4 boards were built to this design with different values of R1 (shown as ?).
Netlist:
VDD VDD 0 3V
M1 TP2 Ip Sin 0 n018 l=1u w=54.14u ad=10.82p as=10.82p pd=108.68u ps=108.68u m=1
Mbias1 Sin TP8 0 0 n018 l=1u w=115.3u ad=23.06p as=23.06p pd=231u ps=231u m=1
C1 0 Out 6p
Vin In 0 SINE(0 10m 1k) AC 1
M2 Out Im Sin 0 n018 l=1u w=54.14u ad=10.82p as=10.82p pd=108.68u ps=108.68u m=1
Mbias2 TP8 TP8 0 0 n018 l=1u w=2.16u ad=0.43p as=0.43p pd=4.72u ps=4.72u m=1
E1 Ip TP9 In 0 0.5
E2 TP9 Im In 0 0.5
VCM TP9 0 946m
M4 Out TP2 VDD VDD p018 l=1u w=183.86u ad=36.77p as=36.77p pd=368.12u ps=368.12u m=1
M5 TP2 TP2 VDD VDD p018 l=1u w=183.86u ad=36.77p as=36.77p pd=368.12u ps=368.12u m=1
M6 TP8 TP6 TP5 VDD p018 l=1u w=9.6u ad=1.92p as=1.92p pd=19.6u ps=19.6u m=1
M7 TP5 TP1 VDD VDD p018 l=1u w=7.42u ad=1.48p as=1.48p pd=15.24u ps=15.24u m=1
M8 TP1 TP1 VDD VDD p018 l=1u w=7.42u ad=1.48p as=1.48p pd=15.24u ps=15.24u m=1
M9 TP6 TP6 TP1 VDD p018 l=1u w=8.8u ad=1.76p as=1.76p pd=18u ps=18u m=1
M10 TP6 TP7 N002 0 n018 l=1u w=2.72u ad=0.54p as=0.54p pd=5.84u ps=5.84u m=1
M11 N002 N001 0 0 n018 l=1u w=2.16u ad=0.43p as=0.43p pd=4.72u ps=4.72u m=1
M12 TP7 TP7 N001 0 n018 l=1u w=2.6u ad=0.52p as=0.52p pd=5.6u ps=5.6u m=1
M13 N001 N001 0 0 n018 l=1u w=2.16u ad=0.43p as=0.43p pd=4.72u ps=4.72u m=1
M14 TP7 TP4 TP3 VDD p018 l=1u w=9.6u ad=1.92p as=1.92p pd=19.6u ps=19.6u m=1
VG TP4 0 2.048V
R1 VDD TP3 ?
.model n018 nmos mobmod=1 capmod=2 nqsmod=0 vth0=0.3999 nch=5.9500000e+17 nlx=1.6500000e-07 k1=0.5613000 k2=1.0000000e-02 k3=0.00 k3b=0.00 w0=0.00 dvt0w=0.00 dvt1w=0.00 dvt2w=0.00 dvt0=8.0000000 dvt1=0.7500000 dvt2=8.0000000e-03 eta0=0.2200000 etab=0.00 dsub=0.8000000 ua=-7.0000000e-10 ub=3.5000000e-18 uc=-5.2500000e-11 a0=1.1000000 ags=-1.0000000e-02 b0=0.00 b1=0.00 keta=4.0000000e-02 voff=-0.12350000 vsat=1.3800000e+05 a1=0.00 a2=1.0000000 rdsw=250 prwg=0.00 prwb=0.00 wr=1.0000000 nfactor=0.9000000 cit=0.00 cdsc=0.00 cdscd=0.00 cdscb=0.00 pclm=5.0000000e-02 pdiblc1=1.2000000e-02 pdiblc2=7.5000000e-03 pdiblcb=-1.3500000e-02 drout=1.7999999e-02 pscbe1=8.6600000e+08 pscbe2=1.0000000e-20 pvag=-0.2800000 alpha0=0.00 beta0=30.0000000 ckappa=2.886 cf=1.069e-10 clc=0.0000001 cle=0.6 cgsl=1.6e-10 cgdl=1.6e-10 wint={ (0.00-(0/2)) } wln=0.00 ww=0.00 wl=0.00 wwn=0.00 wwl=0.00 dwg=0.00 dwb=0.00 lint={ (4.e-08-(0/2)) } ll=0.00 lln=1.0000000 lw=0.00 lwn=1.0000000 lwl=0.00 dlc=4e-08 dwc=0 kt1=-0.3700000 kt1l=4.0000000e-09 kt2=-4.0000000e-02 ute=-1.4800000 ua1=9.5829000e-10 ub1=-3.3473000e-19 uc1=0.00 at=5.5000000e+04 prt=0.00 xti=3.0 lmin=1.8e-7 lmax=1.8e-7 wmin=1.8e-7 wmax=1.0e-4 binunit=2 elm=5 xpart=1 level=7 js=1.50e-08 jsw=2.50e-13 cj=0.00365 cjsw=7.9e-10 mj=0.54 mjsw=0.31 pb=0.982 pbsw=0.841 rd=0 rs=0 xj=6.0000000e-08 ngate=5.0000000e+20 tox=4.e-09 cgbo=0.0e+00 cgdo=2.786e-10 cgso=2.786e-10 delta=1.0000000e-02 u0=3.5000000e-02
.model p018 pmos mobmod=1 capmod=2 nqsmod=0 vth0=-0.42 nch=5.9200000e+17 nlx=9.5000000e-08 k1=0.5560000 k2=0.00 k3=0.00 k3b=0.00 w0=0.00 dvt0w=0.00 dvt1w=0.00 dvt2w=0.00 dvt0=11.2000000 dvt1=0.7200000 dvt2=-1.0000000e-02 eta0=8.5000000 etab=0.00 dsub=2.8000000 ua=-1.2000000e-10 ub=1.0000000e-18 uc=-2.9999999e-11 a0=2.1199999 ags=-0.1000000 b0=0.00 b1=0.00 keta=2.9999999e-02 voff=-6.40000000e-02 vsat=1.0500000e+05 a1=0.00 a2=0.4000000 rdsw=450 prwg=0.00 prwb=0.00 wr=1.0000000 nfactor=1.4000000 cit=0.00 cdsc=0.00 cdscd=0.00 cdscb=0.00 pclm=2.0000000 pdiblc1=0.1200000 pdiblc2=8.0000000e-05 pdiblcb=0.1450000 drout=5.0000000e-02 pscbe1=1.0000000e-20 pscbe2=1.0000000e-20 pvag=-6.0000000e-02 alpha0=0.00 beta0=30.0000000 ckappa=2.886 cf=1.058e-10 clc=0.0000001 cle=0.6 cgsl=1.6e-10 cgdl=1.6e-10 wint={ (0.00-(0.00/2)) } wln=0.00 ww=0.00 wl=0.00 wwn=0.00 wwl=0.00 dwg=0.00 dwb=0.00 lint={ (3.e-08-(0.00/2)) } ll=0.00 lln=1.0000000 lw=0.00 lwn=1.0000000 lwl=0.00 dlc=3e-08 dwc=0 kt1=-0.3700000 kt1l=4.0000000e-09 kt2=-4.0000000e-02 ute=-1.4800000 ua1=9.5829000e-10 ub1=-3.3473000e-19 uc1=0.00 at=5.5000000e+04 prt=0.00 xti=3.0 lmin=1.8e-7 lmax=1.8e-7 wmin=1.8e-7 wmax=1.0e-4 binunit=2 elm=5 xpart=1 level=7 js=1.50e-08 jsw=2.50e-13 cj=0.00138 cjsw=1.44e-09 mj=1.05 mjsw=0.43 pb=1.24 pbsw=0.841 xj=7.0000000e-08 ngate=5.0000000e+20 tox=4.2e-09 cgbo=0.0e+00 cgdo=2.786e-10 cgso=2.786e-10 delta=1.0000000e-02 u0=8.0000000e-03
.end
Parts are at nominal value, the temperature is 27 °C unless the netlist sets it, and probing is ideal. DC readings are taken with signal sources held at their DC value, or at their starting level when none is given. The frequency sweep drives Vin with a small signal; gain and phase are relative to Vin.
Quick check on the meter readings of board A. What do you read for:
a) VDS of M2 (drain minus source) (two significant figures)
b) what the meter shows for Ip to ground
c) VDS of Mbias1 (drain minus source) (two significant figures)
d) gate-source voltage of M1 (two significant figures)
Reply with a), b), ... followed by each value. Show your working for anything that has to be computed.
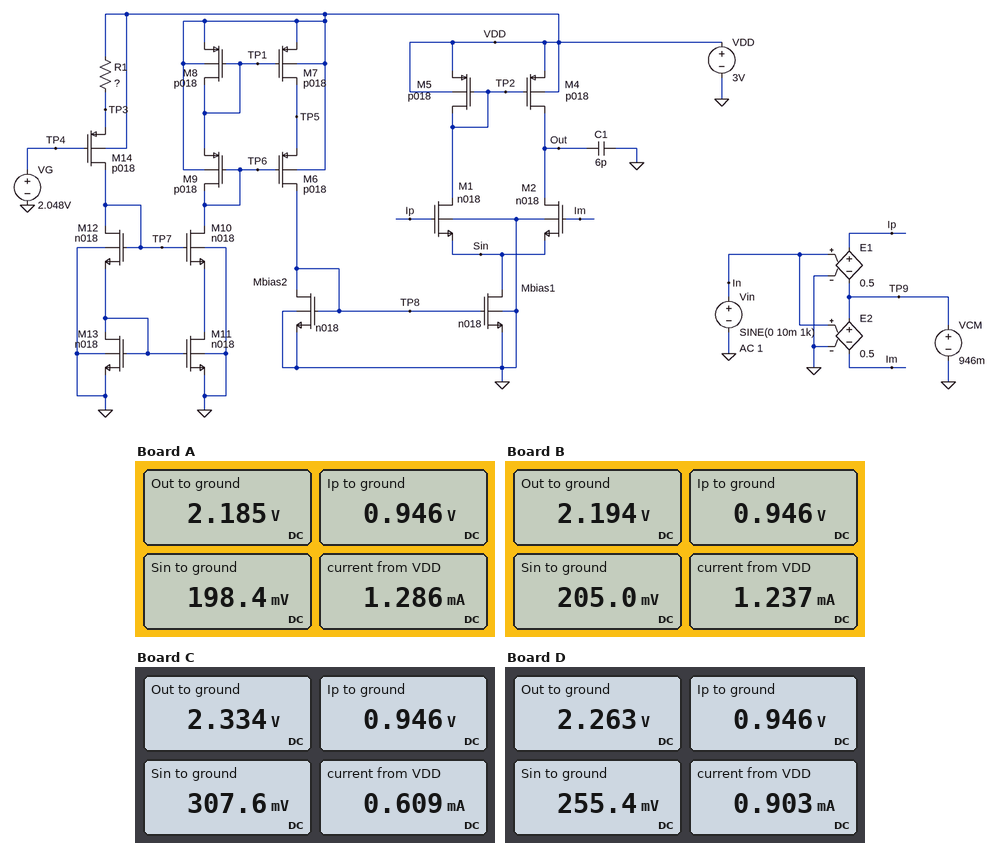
a) 2.185 V - 198.4 mV = 2.0 V
b) 0.946 V
c) 198.4 mV = 200 mV
d) 946 mV - 198.4 mV = 750 mV
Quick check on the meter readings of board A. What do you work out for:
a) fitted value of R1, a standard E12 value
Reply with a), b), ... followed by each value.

a) 6.8 kΩ
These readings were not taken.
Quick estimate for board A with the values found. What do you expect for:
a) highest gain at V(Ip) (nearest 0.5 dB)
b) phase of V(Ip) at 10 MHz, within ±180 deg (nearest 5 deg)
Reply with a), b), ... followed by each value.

a) -6.0 dB
b) 0 deg
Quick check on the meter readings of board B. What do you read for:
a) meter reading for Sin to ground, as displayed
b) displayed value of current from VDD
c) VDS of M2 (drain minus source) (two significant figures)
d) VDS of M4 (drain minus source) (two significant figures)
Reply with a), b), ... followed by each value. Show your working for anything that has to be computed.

a) 205.0 mV
b) 1.237 mA
c) 2.194 V - 205 mV = 2.0 V
d) 2.194 V - 3 V = -810 mV
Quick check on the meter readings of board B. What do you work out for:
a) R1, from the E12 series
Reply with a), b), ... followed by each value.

a) 8.2 kΩ
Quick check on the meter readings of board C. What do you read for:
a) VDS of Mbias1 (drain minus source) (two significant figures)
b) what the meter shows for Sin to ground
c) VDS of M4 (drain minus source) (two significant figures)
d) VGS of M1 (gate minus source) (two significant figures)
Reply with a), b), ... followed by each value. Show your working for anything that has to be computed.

a) 307.6 mV = 310 mV
b) 307.6 mV
c) 2.334 V - 3 V = -670 mV
d) 946 mV - 307.6 mV = 640 mV
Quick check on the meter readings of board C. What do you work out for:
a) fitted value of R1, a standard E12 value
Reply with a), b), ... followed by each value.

a) 47 kΩ
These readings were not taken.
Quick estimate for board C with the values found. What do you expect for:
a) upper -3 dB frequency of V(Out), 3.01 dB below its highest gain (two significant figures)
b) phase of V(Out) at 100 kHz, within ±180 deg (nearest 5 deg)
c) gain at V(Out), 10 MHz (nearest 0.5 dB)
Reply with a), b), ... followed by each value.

a) 1.3 MHz
b) -5 deg
c) 14.0 dB
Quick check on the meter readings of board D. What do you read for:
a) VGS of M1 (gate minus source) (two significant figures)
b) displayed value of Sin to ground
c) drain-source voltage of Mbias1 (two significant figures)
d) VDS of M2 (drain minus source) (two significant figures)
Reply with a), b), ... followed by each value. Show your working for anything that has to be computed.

a) 946 mV - 255.4 mV = 690 mV
b) 255.4 mV
c) 255.4 mV = 260 mV
d) 2.263 V - 255.4 mV = 2.0 V
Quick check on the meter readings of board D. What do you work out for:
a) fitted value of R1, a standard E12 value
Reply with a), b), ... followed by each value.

a) 22 kΩ
